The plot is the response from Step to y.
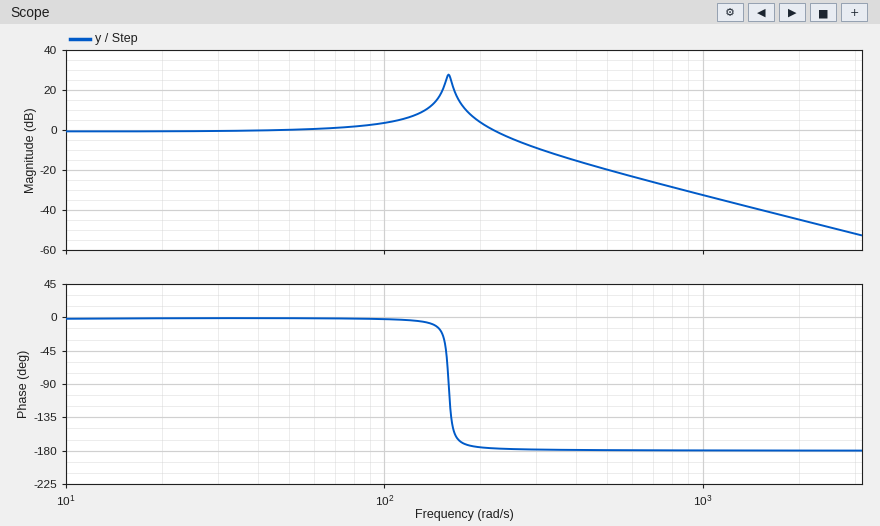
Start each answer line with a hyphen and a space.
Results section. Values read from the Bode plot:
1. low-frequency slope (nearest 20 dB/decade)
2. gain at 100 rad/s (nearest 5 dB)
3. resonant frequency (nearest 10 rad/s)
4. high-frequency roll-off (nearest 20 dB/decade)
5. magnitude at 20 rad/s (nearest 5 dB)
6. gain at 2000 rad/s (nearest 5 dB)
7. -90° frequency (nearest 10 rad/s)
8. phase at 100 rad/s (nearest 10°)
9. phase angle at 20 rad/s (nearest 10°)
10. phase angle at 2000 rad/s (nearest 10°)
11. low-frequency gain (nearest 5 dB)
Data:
- 0 dB/decade
- 5 dB
- 160 rad/s
- -40 dB/decade
- 0 dB
- -45 dB
- 160 rad/s
- 0°
- 0°
- -180°
- 0 dB
